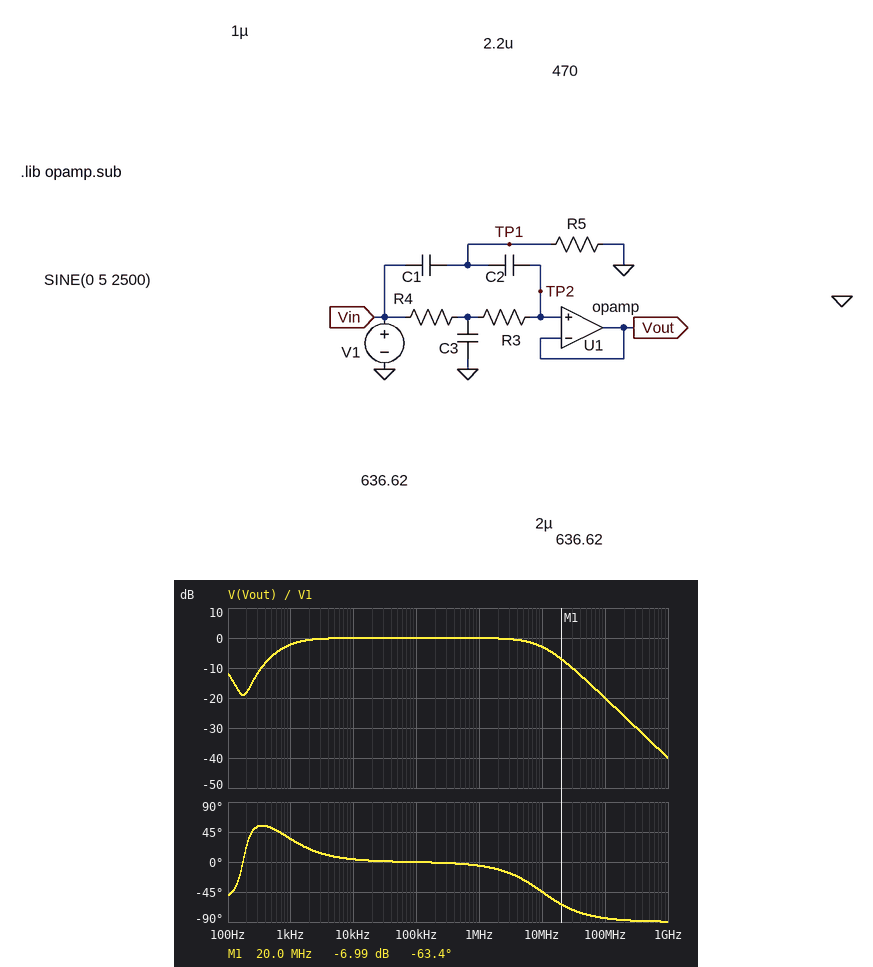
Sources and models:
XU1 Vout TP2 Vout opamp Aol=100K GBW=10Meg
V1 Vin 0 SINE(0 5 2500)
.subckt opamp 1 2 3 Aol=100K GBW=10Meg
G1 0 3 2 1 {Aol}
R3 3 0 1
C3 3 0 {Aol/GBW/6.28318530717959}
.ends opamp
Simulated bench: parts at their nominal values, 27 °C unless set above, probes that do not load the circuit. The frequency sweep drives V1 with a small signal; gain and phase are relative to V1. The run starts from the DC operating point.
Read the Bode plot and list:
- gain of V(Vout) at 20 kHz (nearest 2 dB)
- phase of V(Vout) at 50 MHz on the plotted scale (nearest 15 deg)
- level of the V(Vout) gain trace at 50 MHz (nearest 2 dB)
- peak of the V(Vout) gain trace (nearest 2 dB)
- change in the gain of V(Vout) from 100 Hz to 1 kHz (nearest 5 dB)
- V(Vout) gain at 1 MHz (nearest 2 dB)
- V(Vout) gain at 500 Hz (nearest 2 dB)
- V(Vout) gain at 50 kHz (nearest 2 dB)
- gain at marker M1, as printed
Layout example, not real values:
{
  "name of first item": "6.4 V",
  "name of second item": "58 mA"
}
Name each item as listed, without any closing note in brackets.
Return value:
{
  "gain of V(Vout) at 20 kHz": "0 dB",
  "phase of V(Vout) at 50 MHz on the plotted scale": "-75 deg",
  "level of the V(Vout) gain trace at 50 MHz": "-14 dB",
  "peak of the V(Vout) gain trace": "0 dB",
  "change in the gain of V(Vout) from 100 Hz to 1 kHz": "10 dB",
  "V(Vout) gain at 1 MHz": "0 dB",
  "V(Vout) gain at 500 Hz": "-6 dB",
  "V(Vout) gain at 50 kHz": "0 dB",
  "gain at marker M1, as printed": "-6.99 dB"
}
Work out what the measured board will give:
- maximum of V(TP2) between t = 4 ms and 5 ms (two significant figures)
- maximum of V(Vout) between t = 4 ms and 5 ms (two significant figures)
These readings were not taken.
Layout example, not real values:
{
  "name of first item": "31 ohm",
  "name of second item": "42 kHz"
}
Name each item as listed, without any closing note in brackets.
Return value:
{
  "maximum of V(TP2) between t = 4 ms and 5 ms": "4.8 V",
  "maximum of V(Vout) between t = 4 ms and 5 ms": "4.8 V"
}
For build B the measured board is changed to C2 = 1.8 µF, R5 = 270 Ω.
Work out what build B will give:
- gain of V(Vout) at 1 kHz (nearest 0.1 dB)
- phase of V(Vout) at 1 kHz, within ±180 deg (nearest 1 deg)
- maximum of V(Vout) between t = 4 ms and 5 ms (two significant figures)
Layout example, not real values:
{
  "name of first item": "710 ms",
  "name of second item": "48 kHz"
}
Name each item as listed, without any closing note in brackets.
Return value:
{
  "gain of V(Vout) at 1 kHz": "-3.2 dB",
  "phase of V(Vout) at 1 kHz, within ±180 deg": "45 deg",
  "maximum of V(Vout) between t = 4 ms and 5 ms": "4.7 V"
}
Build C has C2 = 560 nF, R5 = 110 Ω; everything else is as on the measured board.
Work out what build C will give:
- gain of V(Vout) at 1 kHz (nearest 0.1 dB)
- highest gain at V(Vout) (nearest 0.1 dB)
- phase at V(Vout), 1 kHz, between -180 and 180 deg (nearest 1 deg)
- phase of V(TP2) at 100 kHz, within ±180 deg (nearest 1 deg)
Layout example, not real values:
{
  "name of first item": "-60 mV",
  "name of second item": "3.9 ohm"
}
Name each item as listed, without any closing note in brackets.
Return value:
{
  "gain of V(Vout) at 1 kHz": "-7.9 dB",
  "highest gain at V(Vout)": "0 dB",
  "phase at V(Vout), 1 kHz, between -180 and 180 deg": "82 deg",
  "phase of V(TP2) at 100 kHz, within ±180 deg": "1 deg"
}
